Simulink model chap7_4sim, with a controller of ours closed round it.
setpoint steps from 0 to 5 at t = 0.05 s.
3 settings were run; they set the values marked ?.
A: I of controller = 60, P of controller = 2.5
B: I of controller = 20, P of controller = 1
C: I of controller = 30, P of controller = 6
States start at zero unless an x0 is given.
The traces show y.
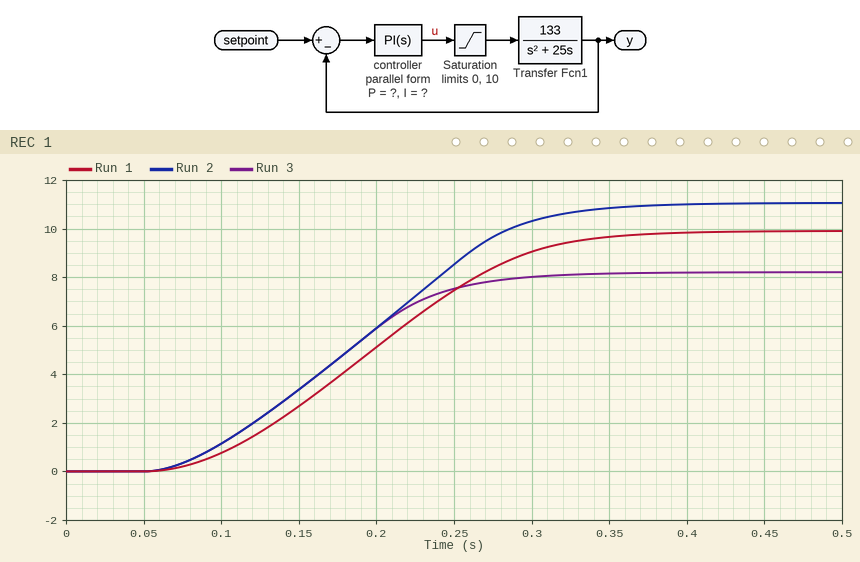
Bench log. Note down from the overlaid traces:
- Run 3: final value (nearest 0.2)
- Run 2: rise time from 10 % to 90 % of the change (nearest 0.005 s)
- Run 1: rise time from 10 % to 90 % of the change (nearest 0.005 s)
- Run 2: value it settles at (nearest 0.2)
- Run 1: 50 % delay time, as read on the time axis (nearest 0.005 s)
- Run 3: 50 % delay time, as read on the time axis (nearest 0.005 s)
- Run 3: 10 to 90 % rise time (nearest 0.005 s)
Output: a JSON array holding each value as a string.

["8.2", "0.185 s", "0.185 s", "11.0", "0.195 s", "0.165 s", "0.150 s"]
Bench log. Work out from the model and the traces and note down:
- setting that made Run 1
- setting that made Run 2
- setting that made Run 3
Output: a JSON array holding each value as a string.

["B", "A", "C"]
